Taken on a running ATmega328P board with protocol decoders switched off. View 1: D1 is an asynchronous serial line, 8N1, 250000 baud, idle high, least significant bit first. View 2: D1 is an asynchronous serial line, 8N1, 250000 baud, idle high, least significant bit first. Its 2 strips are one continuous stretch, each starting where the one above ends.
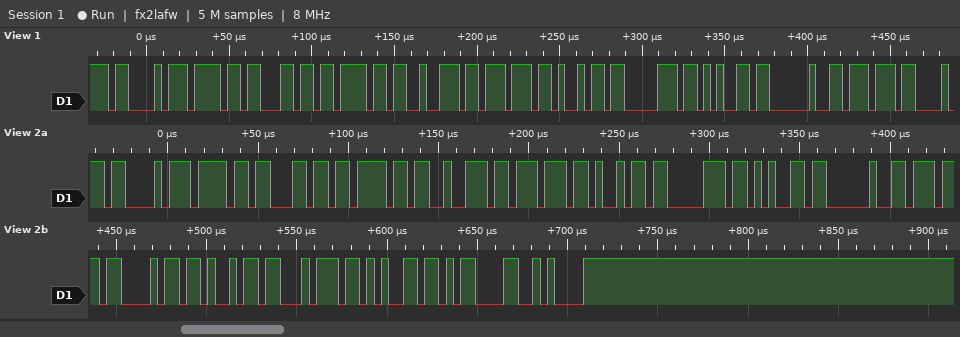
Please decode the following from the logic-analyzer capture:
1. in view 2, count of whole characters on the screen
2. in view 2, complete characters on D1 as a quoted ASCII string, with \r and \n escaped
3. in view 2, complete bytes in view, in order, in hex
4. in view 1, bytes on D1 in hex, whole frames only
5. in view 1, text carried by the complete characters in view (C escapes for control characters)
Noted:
17
"Colorwipe white\r\n"
43 6F 6C 6F 72 77 69 70 65 20 77 68 69 74 65 0D 0A
43 6F 6C 6F 72 77 69 70 65 20 77
"Colorwipe w"
